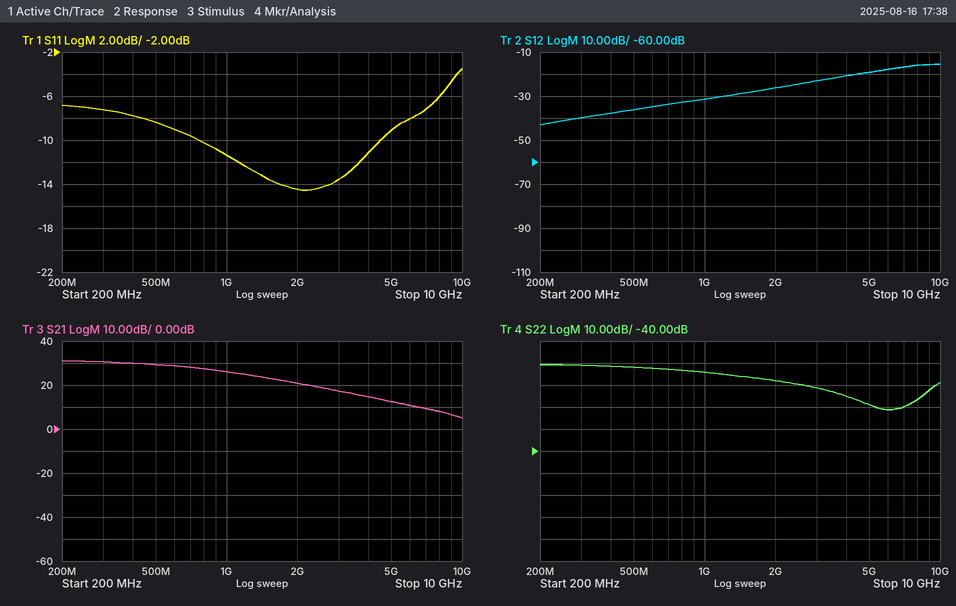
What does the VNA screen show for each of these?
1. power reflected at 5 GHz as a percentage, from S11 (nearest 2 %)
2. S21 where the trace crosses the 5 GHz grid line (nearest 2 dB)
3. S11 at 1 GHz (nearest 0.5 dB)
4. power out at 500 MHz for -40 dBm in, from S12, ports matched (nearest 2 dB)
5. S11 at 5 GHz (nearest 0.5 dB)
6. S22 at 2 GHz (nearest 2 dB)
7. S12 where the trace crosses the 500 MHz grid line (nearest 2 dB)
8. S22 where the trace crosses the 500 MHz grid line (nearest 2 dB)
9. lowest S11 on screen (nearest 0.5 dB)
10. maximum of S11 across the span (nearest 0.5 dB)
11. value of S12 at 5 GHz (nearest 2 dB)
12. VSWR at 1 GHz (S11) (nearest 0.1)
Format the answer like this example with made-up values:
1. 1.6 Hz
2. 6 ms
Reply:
1. 12 %
2. 12 dB
3. -11.5 dB
4. -76 dBm
5. -9.0 dB
6. -8 dB
7. -36 dB
8. -2 dB
9. -14.5 dB
10. -3.5 dB
11. -20 dB
12. 1.7
